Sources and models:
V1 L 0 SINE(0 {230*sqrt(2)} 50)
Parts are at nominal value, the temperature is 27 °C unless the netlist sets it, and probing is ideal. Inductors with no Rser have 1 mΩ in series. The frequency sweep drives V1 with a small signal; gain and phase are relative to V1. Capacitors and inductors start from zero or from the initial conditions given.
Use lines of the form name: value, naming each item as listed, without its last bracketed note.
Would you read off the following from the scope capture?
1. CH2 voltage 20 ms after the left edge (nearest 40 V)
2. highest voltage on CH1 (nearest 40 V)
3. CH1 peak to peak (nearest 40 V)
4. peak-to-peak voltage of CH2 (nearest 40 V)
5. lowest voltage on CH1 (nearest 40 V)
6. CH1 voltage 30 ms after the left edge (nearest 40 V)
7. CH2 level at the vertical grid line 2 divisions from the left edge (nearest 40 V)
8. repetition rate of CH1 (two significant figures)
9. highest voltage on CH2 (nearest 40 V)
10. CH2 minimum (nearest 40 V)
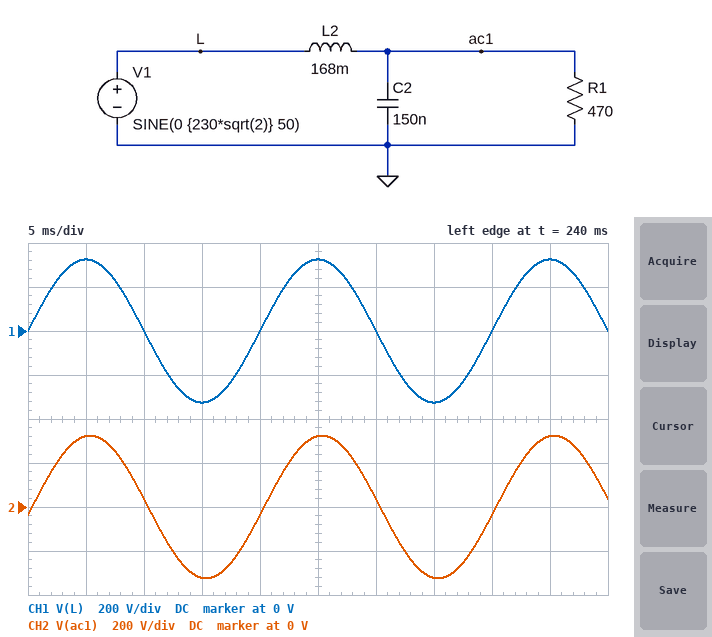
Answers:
CH2 voltage 20 ms after the left edge: -40 V
highest voltage on CH1: 320 V
CH1 peak to peak: 640 V
peak-to-peak voltage of CH2: 640 V
lowest voltage on CH1: -320 V
CH1 voltage 30 ms after the left edge: 0 V
CH2 level at the vertical grid line 2 divisions from the left edge: 40 V
repetition rate of CH1: 50 Hz
highest voltage on CH2: 320 V
CH2 minimum: -320 V
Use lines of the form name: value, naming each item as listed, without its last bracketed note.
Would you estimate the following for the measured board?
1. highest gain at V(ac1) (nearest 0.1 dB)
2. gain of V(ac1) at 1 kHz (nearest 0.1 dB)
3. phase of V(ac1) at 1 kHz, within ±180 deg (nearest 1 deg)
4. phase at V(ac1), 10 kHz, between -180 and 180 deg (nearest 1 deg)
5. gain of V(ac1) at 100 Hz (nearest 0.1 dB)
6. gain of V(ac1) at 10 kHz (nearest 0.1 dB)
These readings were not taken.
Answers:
highest gain at V(ac1): 0 dB
gain of V(ac1) at 1 kHz: -7.0 dB
phase of V(ac1) at 1 kHz, within ±180 deg: -90 deg
phase at V(ac1), 10 kHz, between -180 and 180 deg: -167 deg
gain of V(ac1) at 100 Hz: -0.1 dB
gain of V(ac1) at 10 kHz: -40.1 dB
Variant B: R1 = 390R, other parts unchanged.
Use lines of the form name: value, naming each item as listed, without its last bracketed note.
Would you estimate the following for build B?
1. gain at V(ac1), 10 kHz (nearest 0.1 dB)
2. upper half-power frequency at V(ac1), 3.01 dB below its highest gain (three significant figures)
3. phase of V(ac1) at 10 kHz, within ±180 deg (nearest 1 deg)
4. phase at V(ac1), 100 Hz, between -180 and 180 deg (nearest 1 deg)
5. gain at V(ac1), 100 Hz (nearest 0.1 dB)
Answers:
gain at V(ac1), 10 kHz: -40.2 dB
upper half-power frequency at V(ac1), 3.01 dB below its highest gain: 426 Hz
phase of V(ac1) at 10 kHz, within ±180 deg: -165 deg
phase at V(ac1), 100 Hz, between -180 and 180 deg: -15 deg
gain at V(ac1), 100 Hz: -0.2 dB
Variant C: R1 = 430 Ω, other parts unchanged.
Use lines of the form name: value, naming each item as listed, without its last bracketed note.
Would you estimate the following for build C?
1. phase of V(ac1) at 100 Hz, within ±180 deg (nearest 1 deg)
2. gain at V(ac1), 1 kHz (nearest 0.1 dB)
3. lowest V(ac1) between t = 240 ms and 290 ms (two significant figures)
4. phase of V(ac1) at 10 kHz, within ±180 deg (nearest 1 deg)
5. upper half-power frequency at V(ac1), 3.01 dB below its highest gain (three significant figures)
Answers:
phase of V(ac1) at 100 Hz, within ±180 deg: -14 deg
gain at V(ac1), 1 kHz: -7.8 dB
lowest V(ac1) between t = 240 ms and 290 ms: -320 V
phase of V(ac1) at 10 kHz, within ±180 deg: -166 deg
upper half-power frequency at V(ac1), 3.01 dB below its highest gain: 484 Hz
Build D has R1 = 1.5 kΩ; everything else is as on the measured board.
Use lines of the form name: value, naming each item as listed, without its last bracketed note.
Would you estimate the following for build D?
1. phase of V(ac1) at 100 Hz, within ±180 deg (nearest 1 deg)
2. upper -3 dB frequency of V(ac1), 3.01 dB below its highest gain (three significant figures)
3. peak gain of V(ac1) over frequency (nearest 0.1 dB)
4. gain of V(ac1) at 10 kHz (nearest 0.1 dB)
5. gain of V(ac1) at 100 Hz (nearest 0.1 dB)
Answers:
phase of V(ac1) at 100 Hz, within ±180 deg: -4 deg
upper -3 dB frequency of V(ac1), 3.01 dB below its highest gain: 1.19 kHz
peak gain of V(ac1) over frequency: 3.6 dB
gain of V(ac1) at 10 kHz: -39.9 dB
gain of V(ac1) at 100 Hz: 0.1 dB
